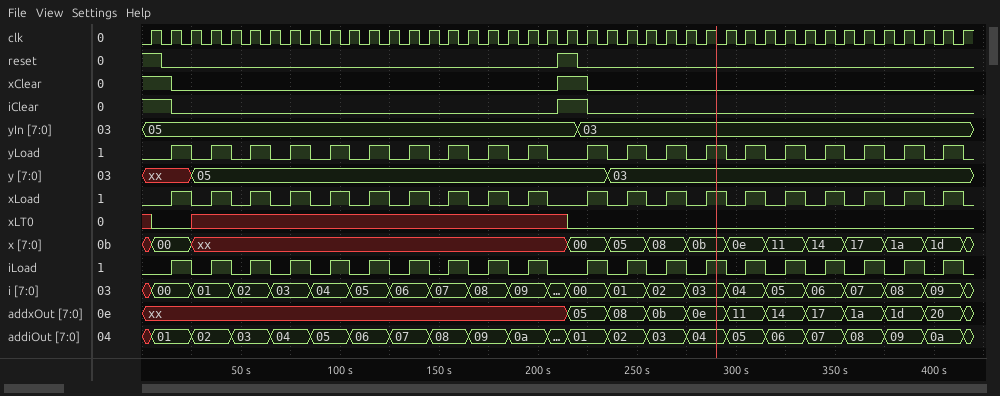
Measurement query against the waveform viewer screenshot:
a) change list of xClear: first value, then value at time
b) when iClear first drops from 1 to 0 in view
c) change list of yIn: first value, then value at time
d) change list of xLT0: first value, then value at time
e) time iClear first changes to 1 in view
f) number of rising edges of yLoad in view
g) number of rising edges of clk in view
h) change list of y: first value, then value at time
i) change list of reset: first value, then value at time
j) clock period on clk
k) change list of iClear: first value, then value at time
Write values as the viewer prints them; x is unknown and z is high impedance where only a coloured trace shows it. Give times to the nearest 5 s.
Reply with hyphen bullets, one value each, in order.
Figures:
- 1, 0 at 15 s, 1 at 210 s, 0 at 225 s
- 15 s
- 05, 03 at 220 s
- x, 0 at 5 s, x at 25 s, 0 at 215 s
- 210 s
- 20
- 42
- xx, 05 at 25 s, 03 at 235 s
- 1, 0 at 10 s, 1 at 210 s, 0 at 220 s
- 10 s
- 1, 0 at 15 s, 1 at 210 s, 0 at 225 s
